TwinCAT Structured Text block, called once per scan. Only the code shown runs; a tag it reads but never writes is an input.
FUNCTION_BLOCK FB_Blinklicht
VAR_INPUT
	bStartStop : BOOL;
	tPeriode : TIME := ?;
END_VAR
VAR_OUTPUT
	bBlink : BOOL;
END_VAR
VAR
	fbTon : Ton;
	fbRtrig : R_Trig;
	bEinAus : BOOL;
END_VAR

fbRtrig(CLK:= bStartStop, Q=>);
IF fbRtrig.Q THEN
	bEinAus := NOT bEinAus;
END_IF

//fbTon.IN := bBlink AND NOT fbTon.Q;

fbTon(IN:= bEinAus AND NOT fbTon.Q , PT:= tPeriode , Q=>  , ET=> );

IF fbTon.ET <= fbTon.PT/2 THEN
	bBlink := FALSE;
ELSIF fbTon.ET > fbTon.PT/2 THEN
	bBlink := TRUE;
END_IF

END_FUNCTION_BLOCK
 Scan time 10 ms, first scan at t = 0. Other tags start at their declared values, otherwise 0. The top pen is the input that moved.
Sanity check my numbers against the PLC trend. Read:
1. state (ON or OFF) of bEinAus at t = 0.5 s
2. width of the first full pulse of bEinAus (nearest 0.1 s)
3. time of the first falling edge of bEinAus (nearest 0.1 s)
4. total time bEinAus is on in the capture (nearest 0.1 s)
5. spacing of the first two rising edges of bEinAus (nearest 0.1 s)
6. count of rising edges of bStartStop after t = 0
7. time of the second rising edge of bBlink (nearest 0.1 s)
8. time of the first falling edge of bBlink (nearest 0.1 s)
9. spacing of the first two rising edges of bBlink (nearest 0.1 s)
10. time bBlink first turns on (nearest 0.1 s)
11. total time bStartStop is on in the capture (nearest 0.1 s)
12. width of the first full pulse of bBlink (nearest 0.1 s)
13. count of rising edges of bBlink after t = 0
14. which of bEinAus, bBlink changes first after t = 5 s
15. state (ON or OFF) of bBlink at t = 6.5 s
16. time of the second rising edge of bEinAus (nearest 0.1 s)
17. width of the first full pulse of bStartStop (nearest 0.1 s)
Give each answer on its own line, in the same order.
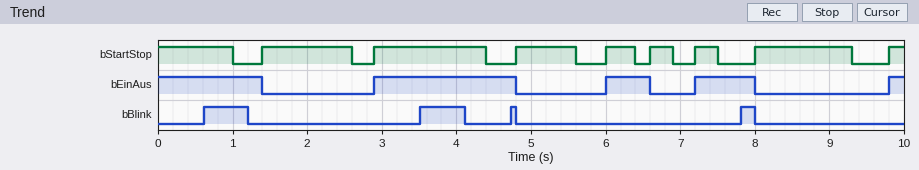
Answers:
ON
1.9 s
1.4 s
4.9 s
3.1 s
8
3.5 s
1.2 s
2.9 s
0.6 s
7.0 s
0.6 s
4
bEinAus
OFF
6.0 s
1.2 s
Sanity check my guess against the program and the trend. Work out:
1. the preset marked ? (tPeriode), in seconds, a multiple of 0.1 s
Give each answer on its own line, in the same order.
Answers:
1.2 s
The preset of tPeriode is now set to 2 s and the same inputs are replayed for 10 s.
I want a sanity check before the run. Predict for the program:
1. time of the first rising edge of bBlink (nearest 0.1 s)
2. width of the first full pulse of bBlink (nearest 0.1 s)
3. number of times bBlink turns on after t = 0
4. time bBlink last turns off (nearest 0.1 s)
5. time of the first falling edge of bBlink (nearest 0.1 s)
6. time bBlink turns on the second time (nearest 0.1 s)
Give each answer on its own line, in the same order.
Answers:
1.0 s
0.4 s
2
4.8 s
1.4 s
3.9 s
